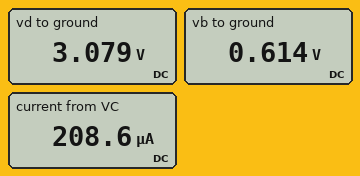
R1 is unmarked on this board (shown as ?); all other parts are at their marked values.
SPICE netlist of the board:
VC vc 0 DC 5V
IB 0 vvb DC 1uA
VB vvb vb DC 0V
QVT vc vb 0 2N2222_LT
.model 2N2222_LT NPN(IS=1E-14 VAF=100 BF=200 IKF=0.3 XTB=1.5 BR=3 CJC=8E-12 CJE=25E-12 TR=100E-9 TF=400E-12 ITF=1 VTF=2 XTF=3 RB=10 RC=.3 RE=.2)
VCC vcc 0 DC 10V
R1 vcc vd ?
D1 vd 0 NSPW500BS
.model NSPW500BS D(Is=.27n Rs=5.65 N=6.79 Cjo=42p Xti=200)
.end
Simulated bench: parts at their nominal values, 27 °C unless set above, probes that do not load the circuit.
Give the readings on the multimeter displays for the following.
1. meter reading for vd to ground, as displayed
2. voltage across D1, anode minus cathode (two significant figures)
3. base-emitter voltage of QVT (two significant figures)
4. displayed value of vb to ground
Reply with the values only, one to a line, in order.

3.079 V
3.1 V
610 mV
0.614 V
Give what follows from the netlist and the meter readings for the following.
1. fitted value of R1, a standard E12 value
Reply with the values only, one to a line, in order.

820 Ω
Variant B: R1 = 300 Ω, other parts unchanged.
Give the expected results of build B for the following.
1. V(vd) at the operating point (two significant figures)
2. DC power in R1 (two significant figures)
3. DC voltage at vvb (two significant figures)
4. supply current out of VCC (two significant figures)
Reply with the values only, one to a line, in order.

3.3 V
150 mW
610 mV
22 mA
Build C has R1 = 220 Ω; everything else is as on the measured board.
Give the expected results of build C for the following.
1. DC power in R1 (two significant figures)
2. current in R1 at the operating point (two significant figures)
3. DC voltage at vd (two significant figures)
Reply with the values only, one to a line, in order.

200 mW
30 mA
3.4 V
